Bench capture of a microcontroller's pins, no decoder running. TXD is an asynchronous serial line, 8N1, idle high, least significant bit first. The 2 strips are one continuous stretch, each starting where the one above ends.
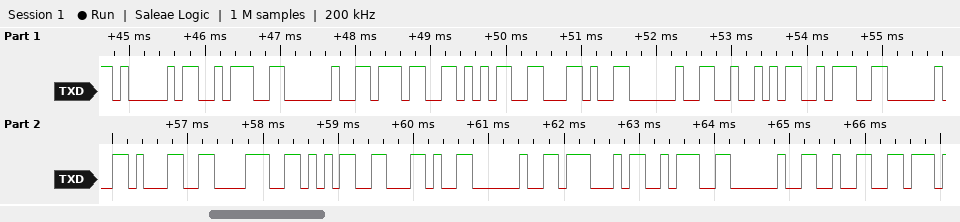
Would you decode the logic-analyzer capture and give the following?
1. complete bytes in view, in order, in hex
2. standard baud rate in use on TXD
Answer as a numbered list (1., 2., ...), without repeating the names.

1. 0x41 0x3A 0x20 0x37 0x35 0x2C 0x20 0x52 0x3A 0x20 0x31 0x38 0x35 0x2C 0x20 0x47 0x3A 0x20 0x32
2. 9600 baud
